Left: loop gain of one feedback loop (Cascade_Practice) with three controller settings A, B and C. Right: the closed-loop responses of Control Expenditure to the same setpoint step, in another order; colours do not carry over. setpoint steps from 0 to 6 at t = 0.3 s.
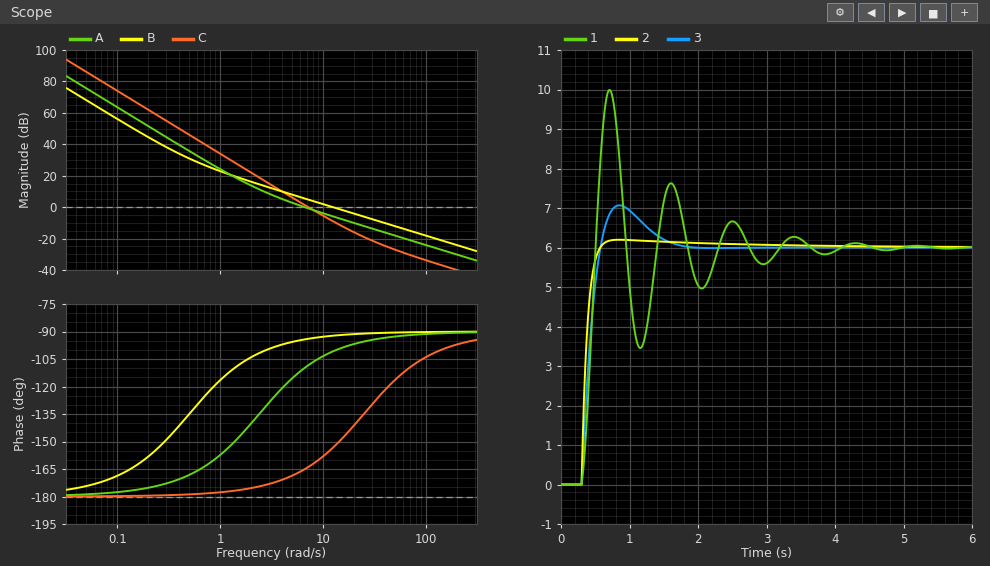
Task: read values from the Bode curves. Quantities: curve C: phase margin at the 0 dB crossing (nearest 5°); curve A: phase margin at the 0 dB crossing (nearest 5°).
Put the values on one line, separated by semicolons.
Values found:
15°; 70°
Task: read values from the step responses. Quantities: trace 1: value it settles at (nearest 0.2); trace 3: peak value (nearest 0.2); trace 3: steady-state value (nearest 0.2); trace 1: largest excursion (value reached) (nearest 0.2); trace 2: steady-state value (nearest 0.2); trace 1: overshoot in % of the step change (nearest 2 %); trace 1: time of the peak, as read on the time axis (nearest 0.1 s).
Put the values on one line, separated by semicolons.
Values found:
6.0; 7.0; 6.0; 10.0; 6.0; 66 %; 0.7 s
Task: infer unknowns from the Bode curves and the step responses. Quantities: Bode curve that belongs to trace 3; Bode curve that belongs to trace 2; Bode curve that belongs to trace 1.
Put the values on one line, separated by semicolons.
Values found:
A; B; C
